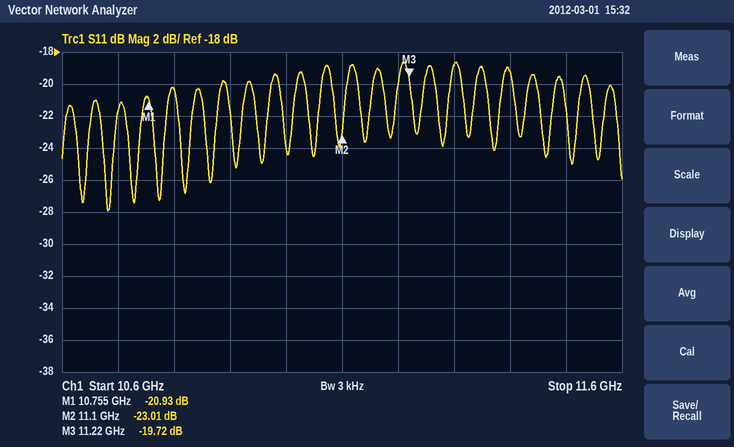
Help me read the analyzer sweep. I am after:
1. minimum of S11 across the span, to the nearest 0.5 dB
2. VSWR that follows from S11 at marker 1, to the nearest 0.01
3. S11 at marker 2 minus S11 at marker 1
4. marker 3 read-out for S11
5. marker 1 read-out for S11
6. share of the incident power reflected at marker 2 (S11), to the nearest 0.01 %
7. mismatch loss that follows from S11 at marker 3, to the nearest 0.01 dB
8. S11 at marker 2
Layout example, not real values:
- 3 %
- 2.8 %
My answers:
- -28.0 dB
- 1.20
- -2.08 dB
- -19.72 dB
- -20.93 dB
- 0.50 %
- 0.05 dB
- -23.01 dB
